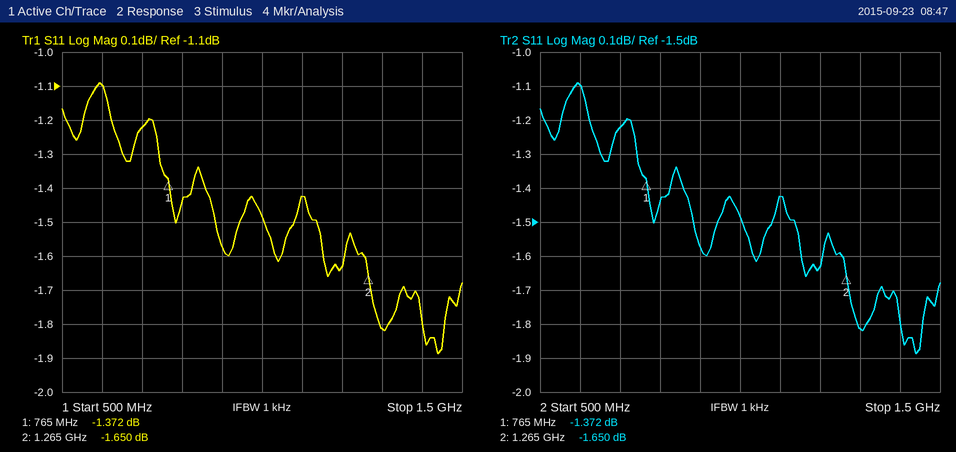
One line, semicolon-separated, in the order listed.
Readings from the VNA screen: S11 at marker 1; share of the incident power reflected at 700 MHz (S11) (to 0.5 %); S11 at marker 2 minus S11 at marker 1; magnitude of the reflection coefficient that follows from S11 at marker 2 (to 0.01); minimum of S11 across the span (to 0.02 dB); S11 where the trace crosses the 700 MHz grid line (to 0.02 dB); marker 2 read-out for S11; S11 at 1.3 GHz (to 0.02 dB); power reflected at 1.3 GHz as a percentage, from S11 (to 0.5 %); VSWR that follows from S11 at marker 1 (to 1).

-1.372 dB; 75.5 %; -0.278 dB; 0.83; -1.88 dB; -1.22 dB; -1.650 dB; -1.82 dB; 66.0 %; 13
